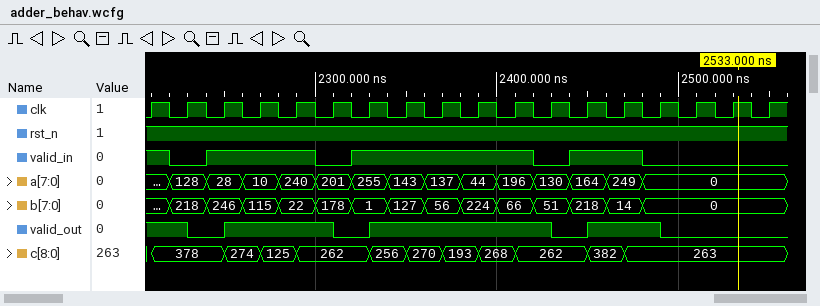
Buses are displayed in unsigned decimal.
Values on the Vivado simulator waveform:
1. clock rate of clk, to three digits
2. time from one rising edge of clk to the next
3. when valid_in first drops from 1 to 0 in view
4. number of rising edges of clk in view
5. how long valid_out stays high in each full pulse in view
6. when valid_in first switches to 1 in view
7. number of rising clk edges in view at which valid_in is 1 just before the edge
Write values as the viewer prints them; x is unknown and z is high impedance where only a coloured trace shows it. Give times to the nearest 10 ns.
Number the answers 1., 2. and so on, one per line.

1. 50.0 MHz
2. 20 ns
3. 2220 ns
4. 18
5. 60 ns, 100 ns, 40 ns
6. 2240 ns
7. 11
